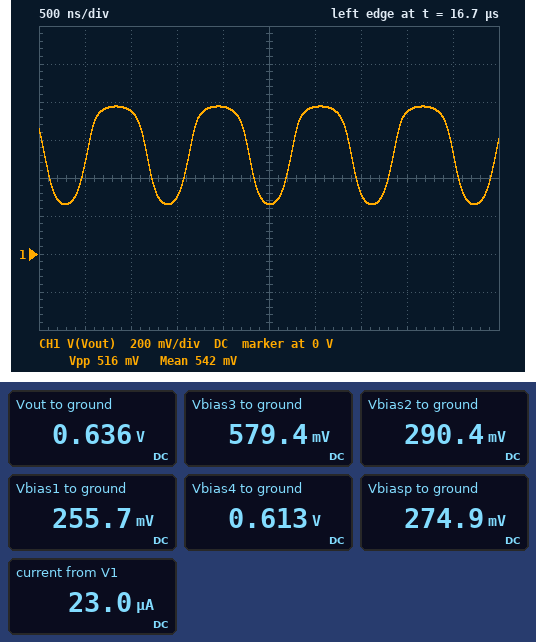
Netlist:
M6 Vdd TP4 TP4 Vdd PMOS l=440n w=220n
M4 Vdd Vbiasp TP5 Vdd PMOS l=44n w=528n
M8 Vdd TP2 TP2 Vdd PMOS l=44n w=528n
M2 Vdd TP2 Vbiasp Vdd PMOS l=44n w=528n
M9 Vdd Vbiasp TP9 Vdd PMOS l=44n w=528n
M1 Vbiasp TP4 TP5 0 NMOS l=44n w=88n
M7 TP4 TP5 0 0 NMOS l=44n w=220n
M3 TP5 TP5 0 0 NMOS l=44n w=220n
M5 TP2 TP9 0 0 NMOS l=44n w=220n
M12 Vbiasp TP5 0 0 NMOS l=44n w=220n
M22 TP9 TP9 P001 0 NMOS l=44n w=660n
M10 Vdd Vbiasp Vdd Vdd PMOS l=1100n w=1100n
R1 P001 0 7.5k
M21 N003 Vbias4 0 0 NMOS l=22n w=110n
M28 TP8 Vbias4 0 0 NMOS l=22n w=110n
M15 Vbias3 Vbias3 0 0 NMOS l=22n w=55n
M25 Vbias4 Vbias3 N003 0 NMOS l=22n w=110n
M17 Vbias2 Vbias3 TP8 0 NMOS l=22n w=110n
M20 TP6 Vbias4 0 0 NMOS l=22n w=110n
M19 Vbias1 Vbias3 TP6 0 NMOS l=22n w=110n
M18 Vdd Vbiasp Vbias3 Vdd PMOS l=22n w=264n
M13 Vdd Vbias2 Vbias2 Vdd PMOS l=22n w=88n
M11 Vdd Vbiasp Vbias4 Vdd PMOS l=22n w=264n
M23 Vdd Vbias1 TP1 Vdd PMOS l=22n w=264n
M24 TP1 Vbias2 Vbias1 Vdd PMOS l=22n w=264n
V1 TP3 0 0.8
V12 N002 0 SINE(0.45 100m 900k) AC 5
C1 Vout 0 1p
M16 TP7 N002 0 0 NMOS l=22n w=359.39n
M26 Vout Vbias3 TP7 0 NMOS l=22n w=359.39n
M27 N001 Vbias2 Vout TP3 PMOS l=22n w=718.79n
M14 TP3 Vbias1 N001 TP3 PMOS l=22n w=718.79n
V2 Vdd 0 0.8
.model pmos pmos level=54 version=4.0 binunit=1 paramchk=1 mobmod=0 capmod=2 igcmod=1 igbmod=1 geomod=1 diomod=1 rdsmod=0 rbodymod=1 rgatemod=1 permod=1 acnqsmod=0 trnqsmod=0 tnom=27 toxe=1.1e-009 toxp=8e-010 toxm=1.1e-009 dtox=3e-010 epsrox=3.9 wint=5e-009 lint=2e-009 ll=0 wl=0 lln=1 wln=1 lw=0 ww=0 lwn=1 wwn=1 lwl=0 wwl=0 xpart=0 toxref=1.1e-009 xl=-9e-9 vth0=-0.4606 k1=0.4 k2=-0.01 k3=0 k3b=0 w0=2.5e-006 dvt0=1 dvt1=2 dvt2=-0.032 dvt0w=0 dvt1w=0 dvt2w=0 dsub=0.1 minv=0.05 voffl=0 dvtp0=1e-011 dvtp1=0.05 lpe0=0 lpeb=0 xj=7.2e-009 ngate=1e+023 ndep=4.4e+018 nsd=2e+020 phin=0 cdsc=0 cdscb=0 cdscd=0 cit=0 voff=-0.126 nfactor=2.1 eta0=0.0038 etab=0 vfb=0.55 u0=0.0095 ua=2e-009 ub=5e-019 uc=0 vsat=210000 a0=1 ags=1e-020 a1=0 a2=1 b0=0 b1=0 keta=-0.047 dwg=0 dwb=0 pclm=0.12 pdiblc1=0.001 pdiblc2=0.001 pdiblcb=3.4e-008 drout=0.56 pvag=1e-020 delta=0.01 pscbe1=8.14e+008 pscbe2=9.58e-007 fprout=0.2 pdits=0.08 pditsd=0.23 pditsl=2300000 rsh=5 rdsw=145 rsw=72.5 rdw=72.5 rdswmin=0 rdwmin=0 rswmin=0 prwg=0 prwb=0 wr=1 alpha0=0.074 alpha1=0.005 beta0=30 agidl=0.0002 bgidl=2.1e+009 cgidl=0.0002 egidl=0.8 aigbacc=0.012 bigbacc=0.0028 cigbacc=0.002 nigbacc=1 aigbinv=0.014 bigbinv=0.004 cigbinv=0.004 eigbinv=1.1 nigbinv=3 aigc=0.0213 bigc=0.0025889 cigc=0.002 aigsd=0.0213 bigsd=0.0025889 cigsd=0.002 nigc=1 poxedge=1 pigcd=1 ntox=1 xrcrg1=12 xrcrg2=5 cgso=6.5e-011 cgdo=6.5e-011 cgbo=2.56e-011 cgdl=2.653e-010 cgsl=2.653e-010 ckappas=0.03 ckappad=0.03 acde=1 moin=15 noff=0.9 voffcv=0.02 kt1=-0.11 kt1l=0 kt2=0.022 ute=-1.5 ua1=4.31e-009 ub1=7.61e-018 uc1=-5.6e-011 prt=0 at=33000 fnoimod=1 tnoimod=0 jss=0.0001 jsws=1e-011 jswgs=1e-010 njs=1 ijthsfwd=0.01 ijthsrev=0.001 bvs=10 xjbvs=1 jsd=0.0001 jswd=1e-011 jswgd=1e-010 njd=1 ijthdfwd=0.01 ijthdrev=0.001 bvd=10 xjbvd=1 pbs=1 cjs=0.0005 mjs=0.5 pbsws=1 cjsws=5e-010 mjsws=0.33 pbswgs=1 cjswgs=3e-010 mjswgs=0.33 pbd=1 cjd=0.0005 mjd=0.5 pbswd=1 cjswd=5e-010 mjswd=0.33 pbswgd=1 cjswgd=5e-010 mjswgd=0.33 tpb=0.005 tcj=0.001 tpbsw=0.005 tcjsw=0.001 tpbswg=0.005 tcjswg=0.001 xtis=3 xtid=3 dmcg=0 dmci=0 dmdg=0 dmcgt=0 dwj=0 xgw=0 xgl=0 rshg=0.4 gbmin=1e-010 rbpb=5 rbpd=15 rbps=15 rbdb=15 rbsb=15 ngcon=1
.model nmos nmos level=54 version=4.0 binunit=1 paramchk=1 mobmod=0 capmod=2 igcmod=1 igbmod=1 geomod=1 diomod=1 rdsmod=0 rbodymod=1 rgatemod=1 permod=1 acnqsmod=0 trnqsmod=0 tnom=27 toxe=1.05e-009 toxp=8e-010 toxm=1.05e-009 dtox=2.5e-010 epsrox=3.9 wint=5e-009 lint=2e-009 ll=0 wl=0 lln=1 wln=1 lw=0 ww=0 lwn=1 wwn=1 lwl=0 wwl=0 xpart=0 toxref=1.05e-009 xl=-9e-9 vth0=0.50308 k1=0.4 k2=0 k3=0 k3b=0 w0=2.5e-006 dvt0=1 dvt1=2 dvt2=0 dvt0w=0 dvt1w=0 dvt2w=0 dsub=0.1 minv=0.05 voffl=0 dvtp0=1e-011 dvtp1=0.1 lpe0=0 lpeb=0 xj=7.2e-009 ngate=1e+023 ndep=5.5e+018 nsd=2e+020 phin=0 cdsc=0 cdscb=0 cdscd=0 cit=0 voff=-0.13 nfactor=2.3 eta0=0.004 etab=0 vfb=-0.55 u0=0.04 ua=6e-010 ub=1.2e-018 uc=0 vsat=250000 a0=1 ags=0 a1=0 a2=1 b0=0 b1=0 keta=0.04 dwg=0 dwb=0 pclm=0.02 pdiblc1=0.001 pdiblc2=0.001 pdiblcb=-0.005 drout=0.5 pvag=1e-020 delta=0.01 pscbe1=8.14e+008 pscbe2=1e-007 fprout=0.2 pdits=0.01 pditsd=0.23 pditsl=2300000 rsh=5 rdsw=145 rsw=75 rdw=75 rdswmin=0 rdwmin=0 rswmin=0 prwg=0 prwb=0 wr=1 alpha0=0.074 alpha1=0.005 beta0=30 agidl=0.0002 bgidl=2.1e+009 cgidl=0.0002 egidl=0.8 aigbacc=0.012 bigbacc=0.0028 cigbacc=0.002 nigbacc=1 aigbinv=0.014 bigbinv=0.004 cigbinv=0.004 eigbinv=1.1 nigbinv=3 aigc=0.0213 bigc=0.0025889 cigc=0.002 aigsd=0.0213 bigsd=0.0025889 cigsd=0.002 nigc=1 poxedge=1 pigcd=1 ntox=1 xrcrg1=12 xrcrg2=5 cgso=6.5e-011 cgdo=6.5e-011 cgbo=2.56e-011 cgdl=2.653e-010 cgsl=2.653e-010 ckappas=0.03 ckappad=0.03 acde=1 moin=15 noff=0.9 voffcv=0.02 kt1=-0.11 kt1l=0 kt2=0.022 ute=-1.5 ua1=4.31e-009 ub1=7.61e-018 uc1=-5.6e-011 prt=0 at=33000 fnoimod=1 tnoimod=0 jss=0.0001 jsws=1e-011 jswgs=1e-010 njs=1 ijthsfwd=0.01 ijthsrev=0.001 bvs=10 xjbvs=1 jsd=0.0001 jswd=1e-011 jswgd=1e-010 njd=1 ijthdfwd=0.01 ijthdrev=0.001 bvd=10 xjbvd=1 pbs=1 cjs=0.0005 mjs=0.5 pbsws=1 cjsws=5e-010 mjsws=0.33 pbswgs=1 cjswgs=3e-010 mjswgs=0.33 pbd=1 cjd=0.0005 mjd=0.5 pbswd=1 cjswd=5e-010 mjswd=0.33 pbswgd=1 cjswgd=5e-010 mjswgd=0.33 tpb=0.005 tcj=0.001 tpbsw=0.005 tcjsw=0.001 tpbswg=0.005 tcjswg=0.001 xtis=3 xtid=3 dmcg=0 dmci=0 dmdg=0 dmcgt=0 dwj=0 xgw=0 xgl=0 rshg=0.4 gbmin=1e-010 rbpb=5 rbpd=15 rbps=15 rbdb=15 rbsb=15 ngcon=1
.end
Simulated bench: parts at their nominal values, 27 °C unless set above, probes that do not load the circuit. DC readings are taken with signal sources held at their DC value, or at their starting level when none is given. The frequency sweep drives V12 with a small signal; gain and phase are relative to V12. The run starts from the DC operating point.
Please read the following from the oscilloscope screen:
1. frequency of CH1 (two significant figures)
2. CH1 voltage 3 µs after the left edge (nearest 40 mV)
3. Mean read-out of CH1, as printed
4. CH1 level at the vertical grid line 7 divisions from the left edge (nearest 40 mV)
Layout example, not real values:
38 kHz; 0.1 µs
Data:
900 kHz; 760 mV; 542 mV; 320 mV
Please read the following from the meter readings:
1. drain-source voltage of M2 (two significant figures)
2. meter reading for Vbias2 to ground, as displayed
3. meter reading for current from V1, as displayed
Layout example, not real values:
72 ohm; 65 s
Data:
530 mV; 290.4 mV; 23.0 µA
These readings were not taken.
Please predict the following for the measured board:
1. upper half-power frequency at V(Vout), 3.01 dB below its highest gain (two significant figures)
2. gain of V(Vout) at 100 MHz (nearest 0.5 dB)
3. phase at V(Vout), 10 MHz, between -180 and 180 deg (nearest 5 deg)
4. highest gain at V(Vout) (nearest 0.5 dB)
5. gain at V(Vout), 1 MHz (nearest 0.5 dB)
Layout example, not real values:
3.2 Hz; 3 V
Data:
13 MHz; -6.5 dB; 145 deg; 11.0 dB; 11.0 dB
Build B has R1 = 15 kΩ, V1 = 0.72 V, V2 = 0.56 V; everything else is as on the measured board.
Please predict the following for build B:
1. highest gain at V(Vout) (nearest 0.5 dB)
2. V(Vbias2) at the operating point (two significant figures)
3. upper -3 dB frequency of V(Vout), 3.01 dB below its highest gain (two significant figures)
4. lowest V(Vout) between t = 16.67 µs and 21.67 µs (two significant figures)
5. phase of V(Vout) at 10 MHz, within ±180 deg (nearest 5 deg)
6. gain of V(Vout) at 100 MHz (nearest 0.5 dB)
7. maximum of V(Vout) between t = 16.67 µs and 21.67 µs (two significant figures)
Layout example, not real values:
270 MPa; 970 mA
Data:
-2.0 dB; 160 mV; 46 MHz; 560 mV; 170 deg; -9.5 dB; 710 mV
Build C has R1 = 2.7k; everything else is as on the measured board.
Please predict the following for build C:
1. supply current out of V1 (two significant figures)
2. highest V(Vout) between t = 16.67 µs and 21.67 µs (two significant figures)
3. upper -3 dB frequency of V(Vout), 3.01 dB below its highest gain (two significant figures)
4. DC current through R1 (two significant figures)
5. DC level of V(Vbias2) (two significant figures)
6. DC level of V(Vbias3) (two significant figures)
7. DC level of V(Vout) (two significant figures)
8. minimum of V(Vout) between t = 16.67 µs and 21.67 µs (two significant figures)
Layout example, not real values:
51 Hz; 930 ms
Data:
29 µA; 780 mV; 30 MHz; 24 µA; 240 mV; 660 mV; 690 mV; 310 mV
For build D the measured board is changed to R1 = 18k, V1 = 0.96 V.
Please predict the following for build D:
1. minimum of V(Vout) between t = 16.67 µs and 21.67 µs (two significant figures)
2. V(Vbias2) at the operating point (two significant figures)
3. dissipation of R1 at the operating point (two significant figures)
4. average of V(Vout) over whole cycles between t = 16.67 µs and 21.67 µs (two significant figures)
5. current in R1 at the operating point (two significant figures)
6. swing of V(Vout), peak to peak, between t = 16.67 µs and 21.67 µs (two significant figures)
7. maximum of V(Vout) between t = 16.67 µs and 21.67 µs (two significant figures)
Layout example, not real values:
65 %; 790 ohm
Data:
800 mV; 330 mV; 110 nW; 890 mV; 2.5 µA; 150 mV; 950 mV
